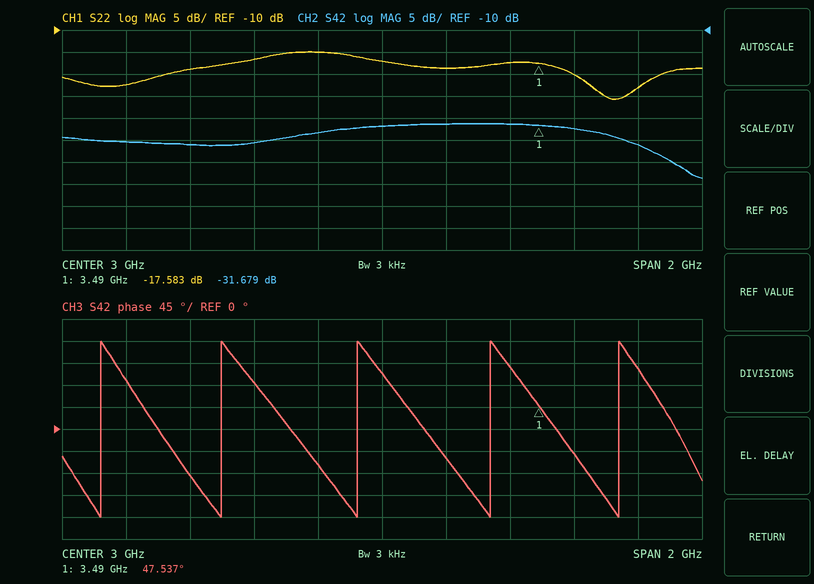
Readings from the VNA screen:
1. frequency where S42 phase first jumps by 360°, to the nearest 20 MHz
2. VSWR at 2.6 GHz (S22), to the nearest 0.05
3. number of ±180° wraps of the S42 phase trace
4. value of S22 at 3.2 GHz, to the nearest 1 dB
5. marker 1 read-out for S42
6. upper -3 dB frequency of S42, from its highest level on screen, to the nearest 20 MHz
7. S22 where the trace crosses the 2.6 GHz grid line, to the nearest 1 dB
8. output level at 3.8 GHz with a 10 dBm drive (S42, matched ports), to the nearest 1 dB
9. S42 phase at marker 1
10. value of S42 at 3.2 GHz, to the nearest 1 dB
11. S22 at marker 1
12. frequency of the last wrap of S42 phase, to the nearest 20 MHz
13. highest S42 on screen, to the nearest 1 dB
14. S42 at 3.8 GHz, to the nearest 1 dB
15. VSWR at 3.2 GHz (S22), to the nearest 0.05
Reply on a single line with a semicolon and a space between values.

2.12 GHz; 1.35; 5; -19 dB; -31.679 dB; 3.72 GHz; -17 dB; -26 dBm; 47.537°; -31 dB; -17.583 dB; 3.74 GHz; -31 dB; -36 dB; 1.25
